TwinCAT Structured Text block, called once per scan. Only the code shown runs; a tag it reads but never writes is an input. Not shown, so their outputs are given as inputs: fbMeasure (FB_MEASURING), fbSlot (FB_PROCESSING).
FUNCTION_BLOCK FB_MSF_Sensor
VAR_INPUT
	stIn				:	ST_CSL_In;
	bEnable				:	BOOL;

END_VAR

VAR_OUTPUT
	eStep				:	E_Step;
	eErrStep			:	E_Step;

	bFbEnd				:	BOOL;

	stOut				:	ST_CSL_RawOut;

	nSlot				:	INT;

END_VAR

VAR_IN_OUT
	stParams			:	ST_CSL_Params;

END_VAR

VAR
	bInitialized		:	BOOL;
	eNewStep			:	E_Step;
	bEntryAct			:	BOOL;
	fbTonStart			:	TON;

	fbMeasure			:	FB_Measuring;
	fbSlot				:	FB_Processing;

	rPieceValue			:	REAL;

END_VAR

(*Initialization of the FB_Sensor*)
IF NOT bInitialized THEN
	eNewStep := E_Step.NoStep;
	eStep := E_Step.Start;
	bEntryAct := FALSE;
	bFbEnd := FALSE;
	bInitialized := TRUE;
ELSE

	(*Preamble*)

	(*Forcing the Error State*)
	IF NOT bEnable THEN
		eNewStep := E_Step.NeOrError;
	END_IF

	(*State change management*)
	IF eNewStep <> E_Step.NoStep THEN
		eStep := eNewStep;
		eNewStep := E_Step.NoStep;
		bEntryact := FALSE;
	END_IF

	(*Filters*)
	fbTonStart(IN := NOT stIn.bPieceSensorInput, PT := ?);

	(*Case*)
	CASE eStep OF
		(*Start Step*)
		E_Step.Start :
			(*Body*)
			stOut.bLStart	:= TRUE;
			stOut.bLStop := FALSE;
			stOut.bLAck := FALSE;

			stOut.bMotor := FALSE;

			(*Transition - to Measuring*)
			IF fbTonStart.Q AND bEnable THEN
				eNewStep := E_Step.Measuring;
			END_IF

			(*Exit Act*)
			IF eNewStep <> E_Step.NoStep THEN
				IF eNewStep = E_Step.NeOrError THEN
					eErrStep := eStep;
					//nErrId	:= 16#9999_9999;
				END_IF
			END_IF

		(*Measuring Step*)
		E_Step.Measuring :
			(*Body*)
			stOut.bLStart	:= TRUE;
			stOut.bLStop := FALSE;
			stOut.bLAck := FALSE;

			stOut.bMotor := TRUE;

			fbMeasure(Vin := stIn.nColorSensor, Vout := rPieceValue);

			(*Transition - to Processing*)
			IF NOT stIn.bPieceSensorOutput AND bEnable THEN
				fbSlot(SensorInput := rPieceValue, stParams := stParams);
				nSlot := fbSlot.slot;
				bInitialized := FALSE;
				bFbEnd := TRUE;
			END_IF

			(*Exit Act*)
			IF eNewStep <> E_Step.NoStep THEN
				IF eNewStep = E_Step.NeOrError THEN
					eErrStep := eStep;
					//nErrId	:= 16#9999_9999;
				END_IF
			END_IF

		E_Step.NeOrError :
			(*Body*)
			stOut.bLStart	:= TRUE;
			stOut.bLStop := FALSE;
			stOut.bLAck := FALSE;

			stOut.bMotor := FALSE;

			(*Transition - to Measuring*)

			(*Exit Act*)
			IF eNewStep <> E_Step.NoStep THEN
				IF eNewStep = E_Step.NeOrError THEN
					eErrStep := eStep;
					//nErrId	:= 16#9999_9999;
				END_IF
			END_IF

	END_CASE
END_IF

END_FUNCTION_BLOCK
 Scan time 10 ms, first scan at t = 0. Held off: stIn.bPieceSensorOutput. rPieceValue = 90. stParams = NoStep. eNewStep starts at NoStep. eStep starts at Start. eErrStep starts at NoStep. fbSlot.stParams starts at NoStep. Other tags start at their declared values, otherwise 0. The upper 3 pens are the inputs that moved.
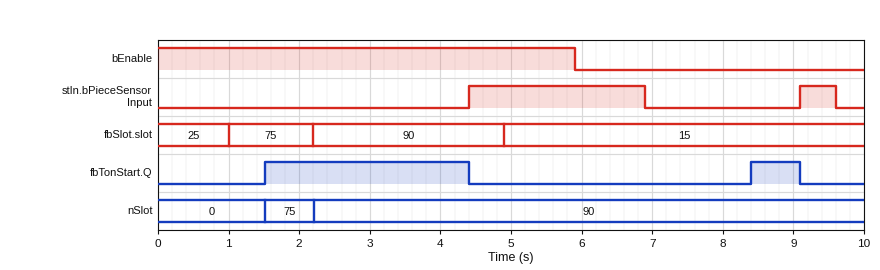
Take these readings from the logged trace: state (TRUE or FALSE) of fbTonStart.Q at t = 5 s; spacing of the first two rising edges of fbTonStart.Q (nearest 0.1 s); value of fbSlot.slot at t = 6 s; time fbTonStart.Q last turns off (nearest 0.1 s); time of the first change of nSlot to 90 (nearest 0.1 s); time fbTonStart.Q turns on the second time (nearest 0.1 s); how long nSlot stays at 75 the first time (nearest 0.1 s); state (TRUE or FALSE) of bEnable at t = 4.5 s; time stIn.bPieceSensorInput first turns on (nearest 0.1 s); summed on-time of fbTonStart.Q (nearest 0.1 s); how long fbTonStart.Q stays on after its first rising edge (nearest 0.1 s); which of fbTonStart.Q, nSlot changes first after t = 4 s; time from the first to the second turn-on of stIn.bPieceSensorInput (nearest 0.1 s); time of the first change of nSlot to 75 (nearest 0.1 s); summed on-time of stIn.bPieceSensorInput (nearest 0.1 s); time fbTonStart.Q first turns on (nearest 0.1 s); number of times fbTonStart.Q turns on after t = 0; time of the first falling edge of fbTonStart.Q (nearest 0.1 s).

FALSE
6.9 s
15
9.1 s
2.2 s
8.4 s
0.7 s
TRUE
4.4 s
3.6 s
2.9 s
fbTonStart.Q
4.7 s
1.5 s
3.0 s
1.5 s
2
4.4 s
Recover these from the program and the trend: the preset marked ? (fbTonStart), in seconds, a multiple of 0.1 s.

1.5 s
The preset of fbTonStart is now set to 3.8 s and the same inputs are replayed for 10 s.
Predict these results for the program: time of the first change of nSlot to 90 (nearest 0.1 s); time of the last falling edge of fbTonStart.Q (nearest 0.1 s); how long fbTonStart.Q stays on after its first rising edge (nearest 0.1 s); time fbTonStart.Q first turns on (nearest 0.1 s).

3.8 s
4.4 s
0.6 s
3.8 s
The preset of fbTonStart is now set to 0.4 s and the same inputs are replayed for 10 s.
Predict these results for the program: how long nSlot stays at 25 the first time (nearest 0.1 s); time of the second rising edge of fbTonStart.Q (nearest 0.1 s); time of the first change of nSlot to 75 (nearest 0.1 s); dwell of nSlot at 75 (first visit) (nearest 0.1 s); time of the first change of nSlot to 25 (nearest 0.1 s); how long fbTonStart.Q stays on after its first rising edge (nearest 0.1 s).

0.6 s
7.3 s
1.0 s
1.2 s
0.4 s
4.0 s
